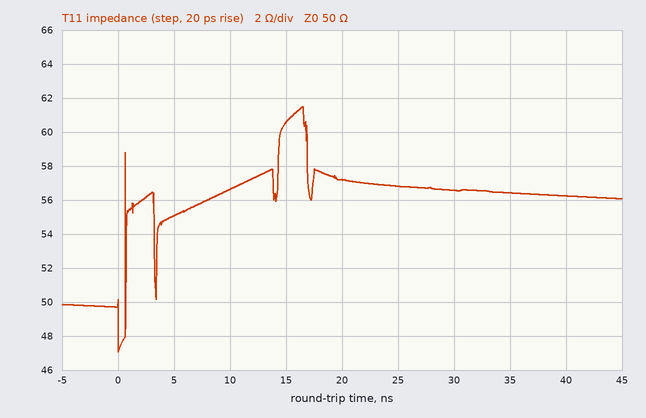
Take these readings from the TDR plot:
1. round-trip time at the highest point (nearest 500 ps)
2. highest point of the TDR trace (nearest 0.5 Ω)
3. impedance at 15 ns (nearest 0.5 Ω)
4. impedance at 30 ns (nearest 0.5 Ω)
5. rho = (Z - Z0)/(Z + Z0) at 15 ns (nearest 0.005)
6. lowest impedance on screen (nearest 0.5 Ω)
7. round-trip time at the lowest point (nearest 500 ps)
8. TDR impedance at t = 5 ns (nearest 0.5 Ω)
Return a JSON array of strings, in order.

["16.5 ns", "61.5 Ω", "60.5 Ω", "56.5 Ω", "+0.095", "47.0 Ω", "0.0 ns", "55.0 Ω"]
